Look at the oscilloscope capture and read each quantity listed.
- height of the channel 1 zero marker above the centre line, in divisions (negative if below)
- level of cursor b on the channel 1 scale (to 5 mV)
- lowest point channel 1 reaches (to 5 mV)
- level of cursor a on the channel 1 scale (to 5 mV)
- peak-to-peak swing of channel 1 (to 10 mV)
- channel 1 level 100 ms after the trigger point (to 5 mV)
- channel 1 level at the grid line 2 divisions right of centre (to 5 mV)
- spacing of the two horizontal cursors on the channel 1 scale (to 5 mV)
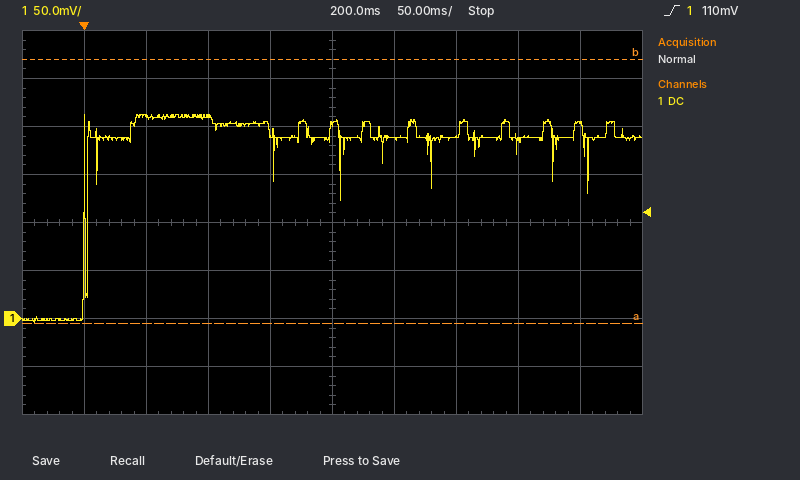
-2.0 div
270 mV
-5 mV
-5 mV
220 mV
210 mV
190 mV
275 mV
